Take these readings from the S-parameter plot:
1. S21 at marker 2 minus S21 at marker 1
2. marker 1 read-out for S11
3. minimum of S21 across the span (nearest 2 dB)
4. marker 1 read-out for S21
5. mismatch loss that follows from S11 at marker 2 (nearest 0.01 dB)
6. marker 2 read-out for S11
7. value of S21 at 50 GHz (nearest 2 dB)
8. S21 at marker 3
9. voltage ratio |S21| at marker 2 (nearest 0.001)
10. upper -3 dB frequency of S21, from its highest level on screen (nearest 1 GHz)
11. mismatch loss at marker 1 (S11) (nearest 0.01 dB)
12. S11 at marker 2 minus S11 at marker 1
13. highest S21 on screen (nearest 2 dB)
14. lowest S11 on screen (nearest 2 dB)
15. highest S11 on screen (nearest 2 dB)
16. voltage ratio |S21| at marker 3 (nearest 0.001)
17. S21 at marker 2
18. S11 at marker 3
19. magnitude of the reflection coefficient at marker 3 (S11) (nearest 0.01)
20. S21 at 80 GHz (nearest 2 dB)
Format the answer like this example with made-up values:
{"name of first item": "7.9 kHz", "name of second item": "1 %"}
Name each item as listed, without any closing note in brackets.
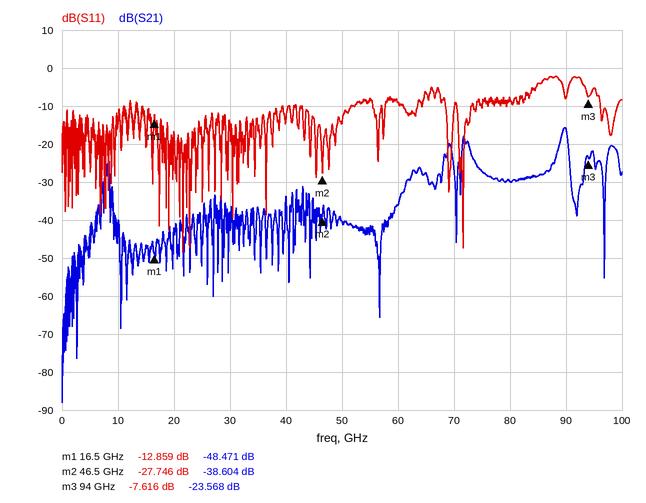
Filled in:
{"S21 at marker 2 minus S21 at marker 1": "9.867 dB", "marker 1 read-out for S11": "-12.859 dB", "minimum of S21 across the span": "-88 dB", "marker 1 read-out for S21": "-48.471 dB", "mismatch loss that follows from S11 at marker 2": "0.01 dB", "marker 2 read-out for S11": "-27.746 dB", "value of S21 at 50 GHz": "-40 dB", "S21 at marker 3": "-23.568 dB", "voltage ratio |S21| at marker 2": "0.012", "upper -3 dB frequency of S21, from its highest level on screen": "90 GHz", "mismatch loss at marker 1 (S11)": "0.23 dB", "S11 at marker 2 minus S11 at marker 1": "-14.887 dB", "highest S21 on screen": "-16 dB", "lowest S11 on screen": "-48 dB", "highest S11 on screen": "-2 dB", "voltage ratio |S21| at marker 3": "0.066", "S21 at marker 2": "-38.604 dB", "S11 at marker 3": "-7.616 dB", "magnitude of the reflection coefficient at marker 3 (S11)": "0.42", "S21 at 80 GHz": "-30 dB"}
